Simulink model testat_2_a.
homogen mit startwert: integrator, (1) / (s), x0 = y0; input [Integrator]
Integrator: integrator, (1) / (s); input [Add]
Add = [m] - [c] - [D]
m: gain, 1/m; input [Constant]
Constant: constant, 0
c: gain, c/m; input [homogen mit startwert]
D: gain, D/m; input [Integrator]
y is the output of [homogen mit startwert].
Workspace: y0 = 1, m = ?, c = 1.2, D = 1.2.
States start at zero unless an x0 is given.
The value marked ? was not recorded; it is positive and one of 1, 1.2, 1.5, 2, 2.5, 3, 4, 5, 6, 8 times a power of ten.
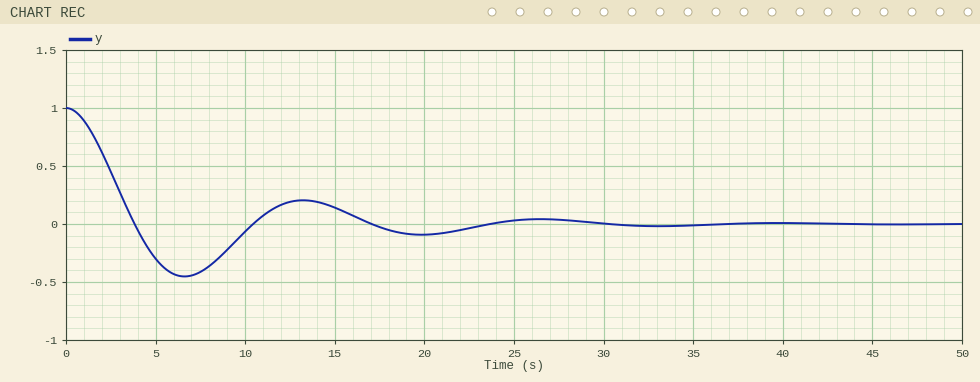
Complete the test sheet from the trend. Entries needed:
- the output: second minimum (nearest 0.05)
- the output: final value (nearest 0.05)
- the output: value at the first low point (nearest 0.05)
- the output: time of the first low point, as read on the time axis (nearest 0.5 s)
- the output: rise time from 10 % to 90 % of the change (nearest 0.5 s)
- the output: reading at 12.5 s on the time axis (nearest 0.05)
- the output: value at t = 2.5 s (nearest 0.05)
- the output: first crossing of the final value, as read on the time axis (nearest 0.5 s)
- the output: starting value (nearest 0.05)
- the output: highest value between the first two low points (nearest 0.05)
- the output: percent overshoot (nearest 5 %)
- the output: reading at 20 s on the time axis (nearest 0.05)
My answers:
-0.10
0.00
-0.45
6.5 s
2.5 s
0.20
0.45
4.0 s
1.00
0.20
45 %
-0.10
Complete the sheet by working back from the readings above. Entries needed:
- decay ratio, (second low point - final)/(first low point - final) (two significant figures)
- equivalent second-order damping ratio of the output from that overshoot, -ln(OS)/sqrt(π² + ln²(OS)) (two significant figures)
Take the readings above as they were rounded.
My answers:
0.22
0.25
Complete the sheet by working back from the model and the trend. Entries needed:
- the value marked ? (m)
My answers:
5
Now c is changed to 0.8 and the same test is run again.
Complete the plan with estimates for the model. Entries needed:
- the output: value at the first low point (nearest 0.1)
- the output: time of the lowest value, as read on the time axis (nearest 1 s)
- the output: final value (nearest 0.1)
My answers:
-0.4
8 s
0.0
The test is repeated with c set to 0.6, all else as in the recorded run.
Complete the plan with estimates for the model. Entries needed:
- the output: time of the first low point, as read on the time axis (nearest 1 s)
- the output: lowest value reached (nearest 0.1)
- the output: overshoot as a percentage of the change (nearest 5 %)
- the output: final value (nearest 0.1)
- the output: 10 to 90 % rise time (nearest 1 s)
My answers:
10 s
-0.3
30 %
0.0
4 s
